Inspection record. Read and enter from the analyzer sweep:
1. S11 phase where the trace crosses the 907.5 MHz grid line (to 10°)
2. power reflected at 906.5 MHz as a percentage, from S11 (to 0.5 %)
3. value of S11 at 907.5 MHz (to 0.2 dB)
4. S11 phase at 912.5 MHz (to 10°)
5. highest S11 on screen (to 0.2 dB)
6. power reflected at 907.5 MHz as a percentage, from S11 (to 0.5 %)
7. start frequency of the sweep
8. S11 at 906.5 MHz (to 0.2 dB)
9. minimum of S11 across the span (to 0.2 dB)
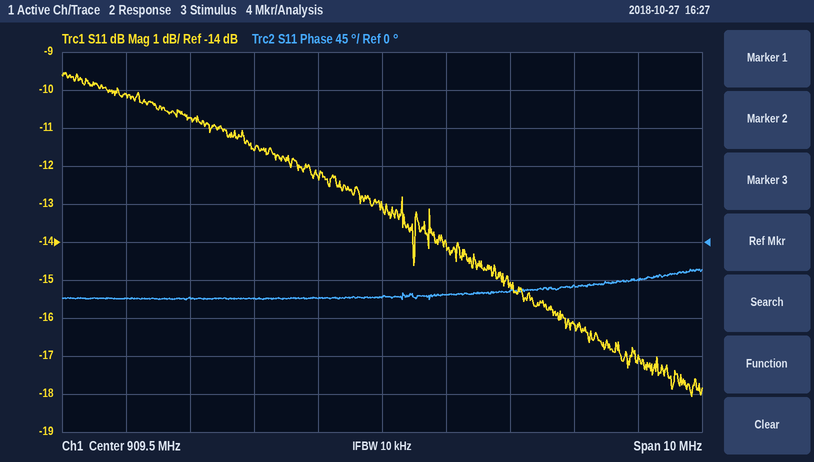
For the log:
-70°
8.5 %
-11.6 dB
-50°
-9.6 dB
7.0 %
904.5 MHz
-10.8 dB
-18.0 dB
